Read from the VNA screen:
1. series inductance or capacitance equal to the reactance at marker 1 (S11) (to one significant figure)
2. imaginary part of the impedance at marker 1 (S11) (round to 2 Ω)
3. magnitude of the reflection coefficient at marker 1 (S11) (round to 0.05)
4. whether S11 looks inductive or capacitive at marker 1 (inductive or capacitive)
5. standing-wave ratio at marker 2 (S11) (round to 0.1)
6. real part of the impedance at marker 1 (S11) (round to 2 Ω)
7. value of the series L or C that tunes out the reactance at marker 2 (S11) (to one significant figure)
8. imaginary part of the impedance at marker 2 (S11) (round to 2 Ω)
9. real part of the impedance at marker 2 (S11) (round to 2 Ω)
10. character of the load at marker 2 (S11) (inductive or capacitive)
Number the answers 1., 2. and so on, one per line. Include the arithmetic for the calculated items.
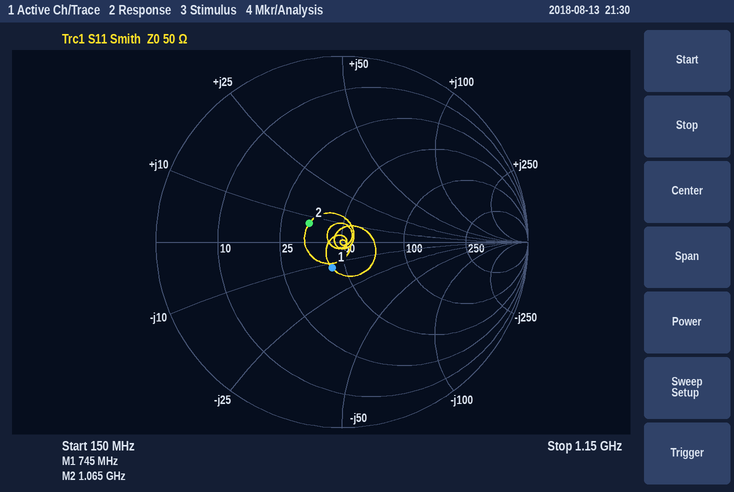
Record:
1. C = 1/(2π × 745 MHz × 12 Ω) ≈ 17.8 pF, so 20 pF to one significant figure
2. -12 Ω
3. 0.15
4. capacitive
5. 1.5
6. 44 Ω
7. C = 1/(2π × 1.065 GHz × 8 Ω) ≈ 18.7 pF, so 20 pF to one significant figure
8. +8 Ω
9. 34 Ω
10. inductive
